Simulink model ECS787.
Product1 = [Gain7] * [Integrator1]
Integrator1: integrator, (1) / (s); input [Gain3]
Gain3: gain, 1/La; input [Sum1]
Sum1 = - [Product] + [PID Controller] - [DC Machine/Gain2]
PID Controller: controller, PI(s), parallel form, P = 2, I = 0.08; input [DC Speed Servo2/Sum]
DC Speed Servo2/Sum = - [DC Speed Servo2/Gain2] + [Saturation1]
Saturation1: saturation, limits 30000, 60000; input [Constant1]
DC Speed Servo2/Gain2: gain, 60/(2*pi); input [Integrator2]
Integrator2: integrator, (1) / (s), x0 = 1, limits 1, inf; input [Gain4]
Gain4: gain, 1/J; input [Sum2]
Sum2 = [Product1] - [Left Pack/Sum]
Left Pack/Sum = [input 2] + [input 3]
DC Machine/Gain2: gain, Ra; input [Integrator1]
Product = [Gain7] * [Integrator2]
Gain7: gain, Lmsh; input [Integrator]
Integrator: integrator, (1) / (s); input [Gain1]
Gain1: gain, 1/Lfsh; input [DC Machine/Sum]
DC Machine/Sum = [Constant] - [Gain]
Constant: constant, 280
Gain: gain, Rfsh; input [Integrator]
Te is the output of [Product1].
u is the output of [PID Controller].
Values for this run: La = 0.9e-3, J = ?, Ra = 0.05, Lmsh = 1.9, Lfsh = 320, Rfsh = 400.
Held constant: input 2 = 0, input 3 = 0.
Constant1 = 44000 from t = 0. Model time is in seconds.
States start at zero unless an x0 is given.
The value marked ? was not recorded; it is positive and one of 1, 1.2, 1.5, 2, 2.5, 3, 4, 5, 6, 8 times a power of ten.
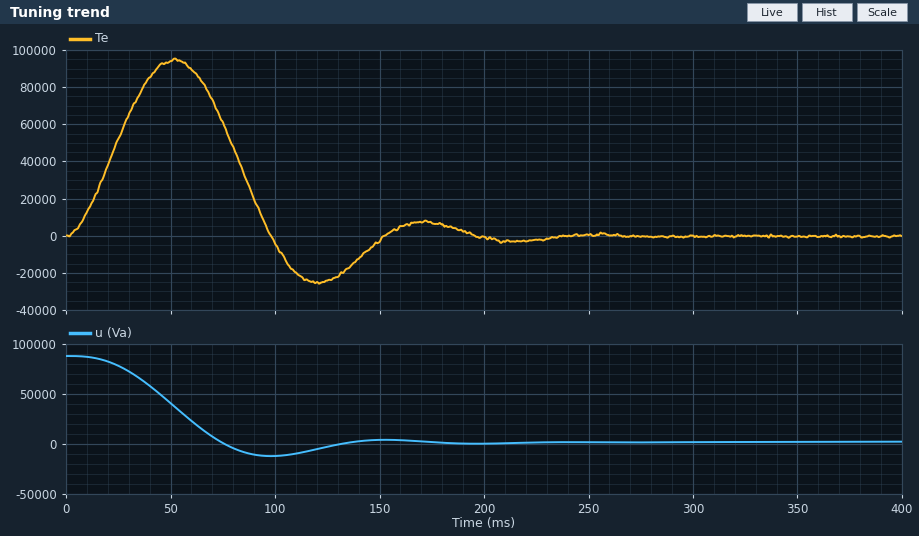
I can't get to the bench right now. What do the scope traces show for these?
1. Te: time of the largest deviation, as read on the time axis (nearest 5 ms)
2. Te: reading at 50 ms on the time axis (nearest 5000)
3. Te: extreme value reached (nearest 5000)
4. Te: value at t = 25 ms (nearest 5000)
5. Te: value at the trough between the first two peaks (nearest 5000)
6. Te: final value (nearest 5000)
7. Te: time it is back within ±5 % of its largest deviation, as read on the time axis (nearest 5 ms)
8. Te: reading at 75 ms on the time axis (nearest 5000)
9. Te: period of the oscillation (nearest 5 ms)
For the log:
50 ms
95000
95000
50000
-25000
0
185 ms
60000
120 ms
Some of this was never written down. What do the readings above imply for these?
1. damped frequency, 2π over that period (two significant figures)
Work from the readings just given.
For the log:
0.052 rad/ms
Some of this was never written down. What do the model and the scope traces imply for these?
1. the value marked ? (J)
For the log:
1
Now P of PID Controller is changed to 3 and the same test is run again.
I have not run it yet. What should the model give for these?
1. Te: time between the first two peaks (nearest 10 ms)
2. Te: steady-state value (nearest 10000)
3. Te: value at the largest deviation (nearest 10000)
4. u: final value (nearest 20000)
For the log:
100 ms
0
120000
0
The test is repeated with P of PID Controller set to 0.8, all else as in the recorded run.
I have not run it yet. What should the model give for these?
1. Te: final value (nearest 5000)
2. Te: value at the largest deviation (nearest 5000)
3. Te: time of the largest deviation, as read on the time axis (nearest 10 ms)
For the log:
0
55000
70 ms
